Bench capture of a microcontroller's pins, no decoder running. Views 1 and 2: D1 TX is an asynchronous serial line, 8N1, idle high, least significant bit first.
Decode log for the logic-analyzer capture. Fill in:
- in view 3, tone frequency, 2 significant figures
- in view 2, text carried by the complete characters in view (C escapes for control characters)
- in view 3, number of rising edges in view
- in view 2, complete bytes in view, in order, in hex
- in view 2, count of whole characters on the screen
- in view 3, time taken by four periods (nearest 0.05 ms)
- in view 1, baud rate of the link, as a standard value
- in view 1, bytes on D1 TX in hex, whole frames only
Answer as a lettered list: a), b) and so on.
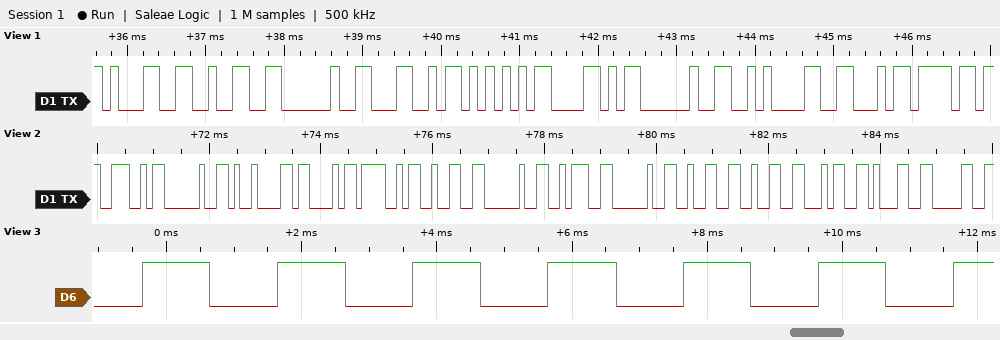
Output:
a) 500 Hz
b) "N \tCO2 : 22410"
c) 7
d) 4E 20 09 43 4F 32 20 3A 20 32 32 34 31 30
e) 14
f) 8.00 ms
g) 9600 baud
h) 0x31 0x32 0x20 0x4C 0x55 0x58 0x20 0x0A 0x46 0x6F
